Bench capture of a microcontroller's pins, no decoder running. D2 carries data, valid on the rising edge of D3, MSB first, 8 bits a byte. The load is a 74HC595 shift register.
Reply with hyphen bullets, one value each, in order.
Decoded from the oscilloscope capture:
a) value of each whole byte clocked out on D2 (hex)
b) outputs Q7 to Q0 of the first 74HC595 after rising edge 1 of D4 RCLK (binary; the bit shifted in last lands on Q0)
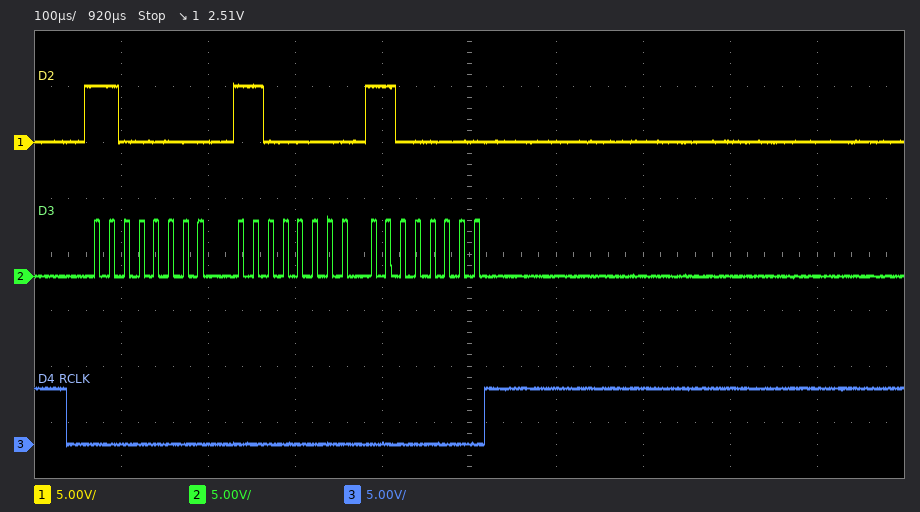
- C0 C0 C0
- 11000000
